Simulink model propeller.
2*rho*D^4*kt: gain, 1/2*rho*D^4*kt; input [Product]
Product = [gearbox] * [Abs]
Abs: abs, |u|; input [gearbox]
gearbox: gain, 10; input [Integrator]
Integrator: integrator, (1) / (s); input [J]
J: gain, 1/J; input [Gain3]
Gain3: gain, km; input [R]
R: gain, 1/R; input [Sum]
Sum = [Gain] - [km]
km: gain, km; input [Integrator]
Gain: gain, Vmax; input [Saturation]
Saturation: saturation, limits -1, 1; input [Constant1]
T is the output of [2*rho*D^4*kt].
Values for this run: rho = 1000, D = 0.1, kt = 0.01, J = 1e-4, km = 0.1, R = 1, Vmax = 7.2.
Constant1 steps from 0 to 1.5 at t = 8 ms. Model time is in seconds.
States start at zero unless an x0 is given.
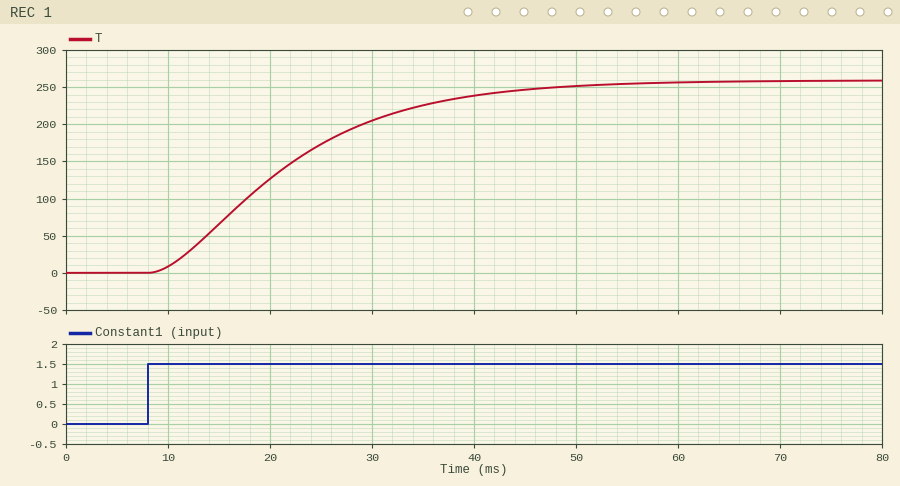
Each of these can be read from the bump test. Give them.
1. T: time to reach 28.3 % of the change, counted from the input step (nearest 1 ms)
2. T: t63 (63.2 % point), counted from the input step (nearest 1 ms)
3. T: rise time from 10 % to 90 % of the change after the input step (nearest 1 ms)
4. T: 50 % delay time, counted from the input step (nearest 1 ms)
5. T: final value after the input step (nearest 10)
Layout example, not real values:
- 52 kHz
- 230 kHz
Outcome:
- 8 ms
- 16 ms
- 26 ms
- 12 ms
- 260
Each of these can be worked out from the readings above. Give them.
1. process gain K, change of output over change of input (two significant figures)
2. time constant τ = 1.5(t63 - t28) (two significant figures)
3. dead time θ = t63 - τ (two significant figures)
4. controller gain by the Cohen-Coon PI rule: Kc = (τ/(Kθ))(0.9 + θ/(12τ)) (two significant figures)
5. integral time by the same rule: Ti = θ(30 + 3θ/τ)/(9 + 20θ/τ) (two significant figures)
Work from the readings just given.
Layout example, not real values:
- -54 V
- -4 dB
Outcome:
- 170
- 12 ms
- 4.0 ms
- 0.016
- 7.9 ms
